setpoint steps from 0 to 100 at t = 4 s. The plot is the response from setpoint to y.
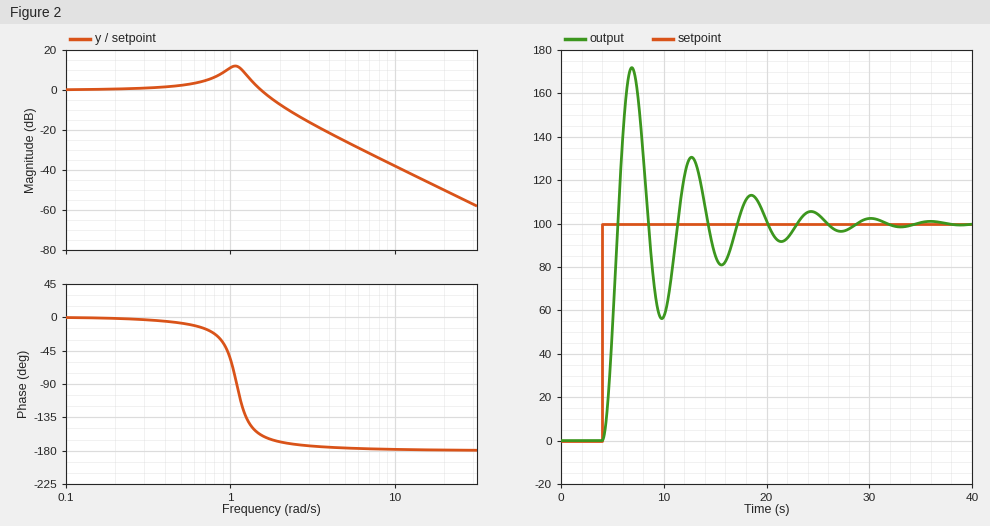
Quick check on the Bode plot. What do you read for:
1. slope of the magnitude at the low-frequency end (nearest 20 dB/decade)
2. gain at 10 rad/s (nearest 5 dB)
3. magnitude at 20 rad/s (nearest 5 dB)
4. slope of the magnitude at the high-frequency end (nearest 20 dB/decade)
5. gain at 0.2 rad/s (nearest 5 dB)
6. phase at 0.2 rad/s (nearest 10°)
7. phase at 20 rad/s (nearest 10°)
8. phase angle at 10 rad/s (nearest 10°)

0 dB/decade
-40 dB
-50 dB
-40 dB/decade
0 dB
0°
-180°
-180°
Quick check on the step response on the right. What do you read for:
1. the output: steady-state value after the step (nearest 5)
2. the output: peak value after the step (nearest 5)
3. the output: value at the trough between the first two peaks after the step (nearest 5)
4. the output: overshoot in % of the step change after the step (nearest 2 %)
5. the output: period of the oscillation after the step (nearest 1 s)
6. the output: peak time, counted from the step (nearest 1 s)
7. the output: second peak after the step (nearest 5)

100
170
55
72 %
6 s
3 s
130
